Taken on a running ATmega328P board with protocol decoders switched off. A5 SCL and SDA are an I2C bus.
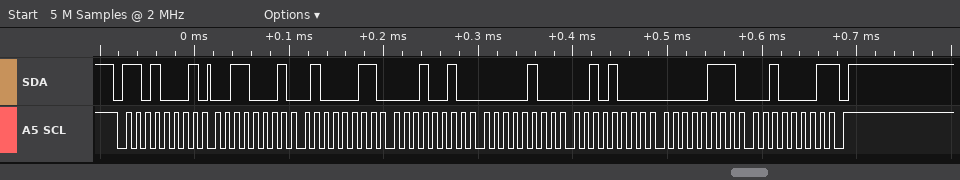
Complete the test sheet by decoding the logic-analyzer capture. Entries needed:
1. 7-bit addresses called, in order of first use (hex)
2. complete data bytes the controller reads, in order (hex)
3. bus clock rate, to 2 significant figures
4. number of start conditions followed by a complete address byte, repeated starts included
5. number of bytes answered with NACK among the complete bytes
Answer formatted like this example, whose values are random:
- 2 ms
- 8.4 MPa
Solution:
- 0x68
- 31 43 12 04 28 07 21
- 100 kHz
- 1
- 1
